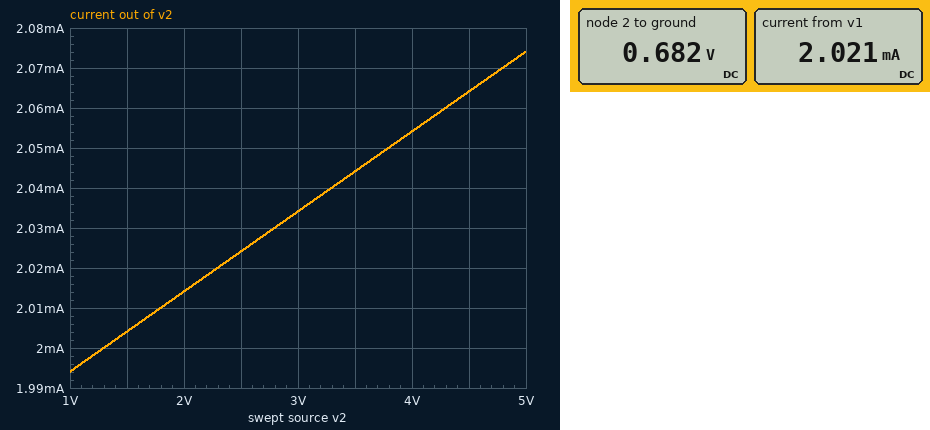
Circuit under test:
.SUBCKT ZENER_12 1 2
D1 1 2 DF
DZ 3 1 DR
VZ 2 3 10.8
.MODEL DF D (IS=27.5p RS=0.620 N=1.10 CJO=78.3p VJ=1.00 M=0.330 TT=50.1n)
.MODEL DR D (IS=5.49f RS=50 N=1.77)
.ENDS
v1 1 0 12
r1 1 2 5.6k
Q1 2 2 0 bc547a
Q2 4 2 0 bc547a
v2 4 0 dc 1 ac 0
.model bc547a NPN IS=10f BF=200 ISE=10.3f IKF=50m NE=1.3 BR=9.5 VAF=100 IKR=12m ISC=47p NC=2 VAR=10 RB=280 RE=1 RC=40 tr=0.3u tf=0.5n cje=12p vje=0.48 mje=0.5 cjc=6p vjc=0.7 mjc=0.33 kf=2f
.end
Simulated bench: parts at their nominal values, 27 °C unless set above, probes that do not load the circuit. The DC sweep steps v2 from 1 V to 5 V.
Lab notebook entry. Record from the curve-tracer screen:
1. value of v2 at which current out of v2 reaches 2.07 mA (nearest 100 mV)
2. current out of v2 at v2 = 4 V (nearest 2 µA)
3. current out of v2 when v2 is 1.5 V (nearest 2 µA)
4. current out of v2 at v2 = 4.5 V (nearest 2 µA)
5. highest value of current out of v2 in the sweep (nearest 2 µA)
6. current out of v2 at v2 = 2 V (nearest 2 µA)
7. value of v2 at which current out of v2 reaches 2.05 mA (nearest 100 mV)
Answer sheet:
4.8 V
2.054 mA
2.004 mA
2.064 mA
2.074 mA
2.014 mA
3.8 V
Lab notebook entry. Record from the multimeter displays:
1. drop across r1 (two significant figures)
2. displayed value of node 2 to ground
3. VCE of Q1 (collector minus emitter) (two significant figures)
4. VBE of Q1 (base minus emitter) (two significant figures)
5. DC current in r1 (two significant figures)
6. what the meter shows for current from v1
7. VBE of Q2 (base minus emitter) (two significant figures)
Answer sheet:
11 V
0.682 V
680 mV
680 mV
2.0 mA
2.021 mA
680 mV
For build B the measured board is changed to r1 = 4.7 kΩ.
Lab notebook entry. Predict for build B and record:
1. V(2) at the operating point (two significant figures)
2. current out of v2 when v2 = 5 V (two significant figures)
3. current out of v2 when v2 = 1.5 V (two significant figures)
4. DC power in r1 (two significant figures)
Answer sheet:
690 mV
2.5 mA
2.4 mA
27 mW
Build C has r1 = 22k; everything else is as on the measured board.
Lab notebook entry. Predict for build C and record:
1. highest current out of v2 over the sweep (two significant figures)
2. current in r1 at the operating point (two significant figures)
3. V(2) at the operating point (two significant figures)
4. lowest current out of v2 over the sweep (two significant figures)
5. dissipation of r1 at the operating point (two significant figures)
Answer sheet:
530 µA
520 µA
640 mV
510 µA
5.9 mW
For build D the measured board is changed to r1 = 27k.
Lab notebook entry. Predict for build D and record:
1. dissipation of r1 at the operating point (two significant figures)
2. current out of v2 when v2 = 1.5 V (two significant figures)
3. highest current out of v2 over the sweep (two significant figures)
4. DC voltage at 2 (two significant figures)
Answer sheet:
4.8 mW
420 µA
430 µA
640 mV
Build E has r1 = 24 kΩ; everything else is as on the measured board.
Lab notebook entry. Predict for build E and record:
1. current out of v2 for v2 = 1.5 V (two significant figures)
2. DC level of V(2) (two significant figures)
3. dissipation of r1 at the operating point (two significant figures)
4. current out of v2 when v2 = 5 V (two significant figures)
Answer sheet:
470 µA
640 mV
5.4 mW
490 µA
